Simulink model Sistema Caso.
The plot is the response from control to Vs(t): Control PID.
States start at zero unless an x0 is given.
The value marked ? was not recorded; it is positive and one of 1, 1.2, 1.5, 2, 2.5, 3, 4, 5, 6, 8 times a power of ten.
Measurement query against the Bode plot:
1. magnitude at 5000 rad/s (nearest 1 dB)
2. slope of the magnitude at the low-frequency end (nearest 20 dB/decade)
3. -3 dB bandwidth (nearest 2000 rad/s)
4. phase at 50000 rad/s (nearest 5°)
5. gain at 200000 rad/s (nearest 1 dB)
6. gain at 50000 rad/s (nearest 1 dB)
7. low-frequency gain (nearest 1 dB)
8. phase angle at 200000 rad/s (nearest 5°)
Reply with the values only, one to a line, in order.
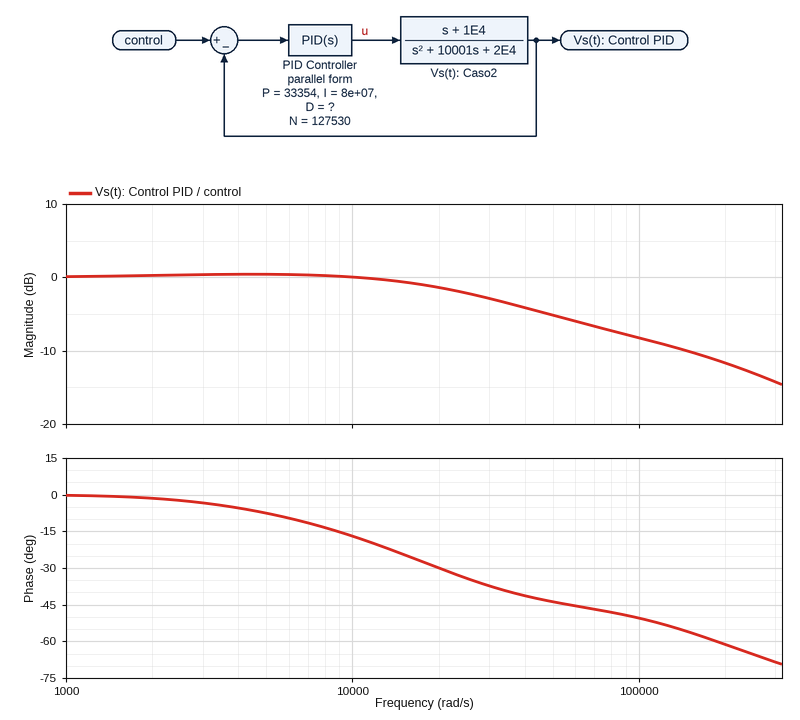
0 dB
0 dB/decade
30000 rad/s
-45°
-12 dB
-5 dB
0 dB
-60°
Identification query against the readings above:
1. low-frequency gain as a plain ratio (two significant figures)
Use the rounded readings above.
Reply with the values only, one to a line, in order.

1.0
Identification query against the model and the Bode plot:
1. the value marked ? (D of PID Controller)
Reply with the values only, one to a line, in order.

0.25
